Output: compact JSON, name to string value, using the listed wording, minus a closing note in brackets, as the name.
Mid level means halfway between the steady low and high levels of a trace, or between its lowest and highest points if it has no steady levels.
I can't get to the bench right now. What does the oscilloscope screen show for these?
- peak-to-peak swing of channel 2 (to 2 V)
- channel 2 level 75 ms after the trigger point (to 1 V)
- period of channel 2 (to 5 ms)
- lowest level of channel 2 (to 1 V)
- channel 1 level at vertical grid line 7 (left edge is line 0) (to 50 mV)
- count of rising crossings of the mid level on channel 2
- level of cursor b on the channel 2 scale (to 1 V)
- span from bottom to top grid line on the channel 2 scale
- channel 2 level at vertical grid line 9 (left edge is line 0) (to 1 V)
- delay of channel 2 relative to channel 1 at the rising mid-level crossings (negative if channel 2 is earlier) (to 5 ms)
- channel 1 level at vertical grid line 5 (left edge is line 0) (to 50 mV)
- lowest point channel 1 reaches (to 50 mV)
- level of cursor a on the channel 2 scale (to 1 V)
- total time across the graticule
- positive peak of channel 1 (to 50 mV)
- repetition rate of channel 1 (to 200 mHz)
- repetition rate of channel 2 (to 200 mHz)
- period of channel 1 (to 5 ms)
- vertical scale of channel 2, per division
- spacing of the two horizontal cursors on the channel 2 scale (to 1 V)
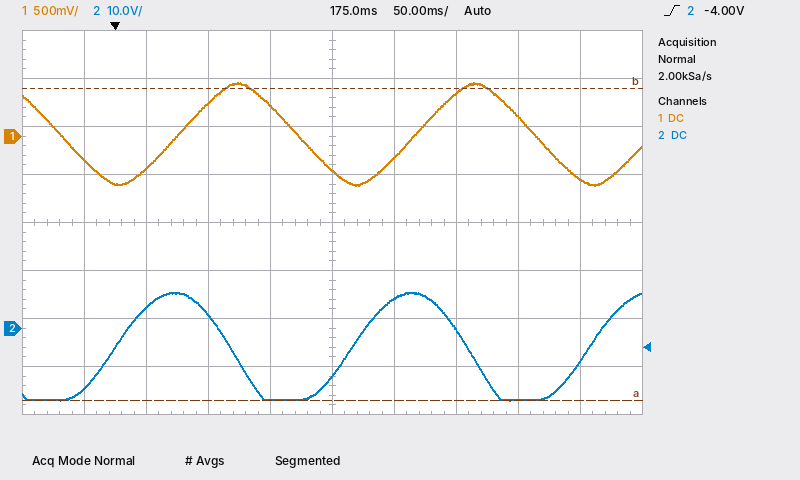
{"peak-to-peak swing of channel 2": "22 V", "channel 2 level 75 ms after the trigger point": "3 V", "period of channel 2": "190 ms", "lowest level of channel 2": "-15 V", "channel 1 level at vertical grid line 7 (left edge is line 0)": "450 mV", "count of rising crossings of the mid level on channel 2": "3", "level of cursor b on the channel 2 scale": "50 V", "span from bottom to top grid line on the channel 2 scale": "80 V", "channel 2 level at vertical grid line 9 (left edge is line 0)": "-7 V", "delay of channel 2 relative to channel 1 at the rising mid-level crossings (negative if channel 2 is earlier)": "-50 ms", "channel 1 level at vertical grid line 5 (left edge is line 0)": "-350 mV", "lowest point channel 1 reaches": "-500 mV", "level of cursor a on the channel 2 scale": "-15 V", "total time across the graticule": "500 ms", "positive peak of channel 1": "550 mV", "repetition rate of channel 1": "5.2 Hz", "repetition rate of channel 2": "5.2 Hz", "period of channel 1": "190 ms", "vertical scale of channel 2, per division": "10 V", "spacing of the two horizontal cursors on the channel 2 scale": "65 V"}
